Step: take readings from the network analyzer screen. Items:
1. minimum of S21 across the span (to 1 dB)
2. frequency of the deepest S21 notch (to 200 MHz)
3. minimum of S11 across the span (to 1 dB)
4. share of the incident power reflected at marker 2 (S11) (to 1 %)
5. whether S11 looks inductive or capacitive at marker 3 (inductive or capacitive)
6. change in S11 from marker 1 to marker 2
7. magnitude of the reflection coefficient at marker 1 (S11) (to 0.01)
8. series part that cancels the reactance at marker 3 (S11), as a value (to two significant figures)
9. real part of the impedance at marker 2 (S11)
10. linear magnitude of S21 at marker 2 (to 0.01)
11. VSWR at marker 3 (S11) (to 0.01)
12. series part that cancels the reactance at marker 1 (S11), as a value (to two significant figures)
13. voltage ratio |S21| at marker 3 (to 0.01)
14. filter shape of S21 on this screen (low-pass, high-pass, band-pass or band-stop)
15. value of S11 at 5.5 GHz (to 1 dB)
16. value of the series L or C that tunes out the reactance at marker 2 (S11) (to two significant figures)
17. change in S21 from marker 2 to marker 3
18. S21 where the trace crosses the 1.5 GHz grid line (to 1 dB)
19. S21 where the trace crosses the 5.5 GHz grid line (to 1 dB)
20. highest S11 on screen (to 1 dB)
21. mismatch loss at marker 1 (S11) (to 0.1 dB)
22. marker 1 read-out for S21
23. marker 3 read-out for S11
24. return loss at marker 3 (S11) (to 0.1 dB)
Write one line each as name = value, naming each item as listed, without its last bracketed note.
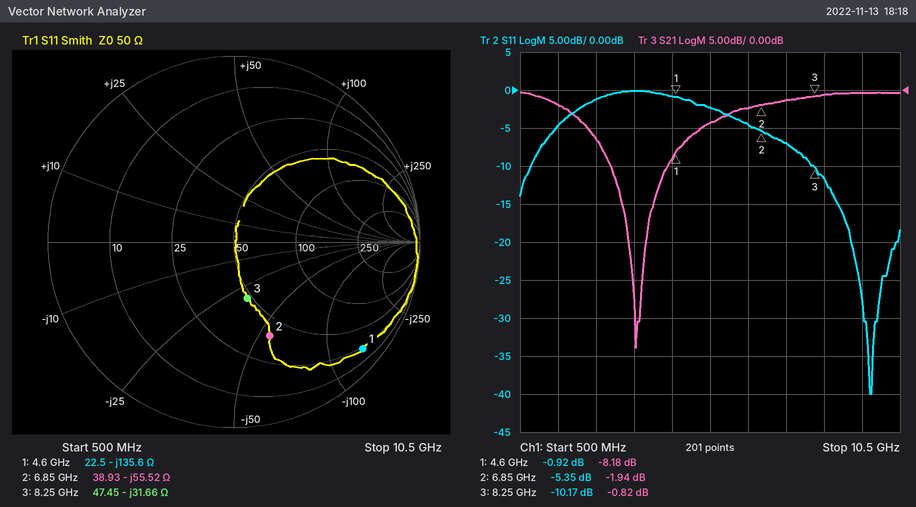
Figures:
minimum of S21 across the span = -34 dB
frequency of the deepest S21 notch = 3.6 GHz
minimum of S11 across the span = -40 dB
share of the incident power reflected at marker 2 (S11) = 29 %
whether S11 looks inductive or capacitive at marker 3 = capacitive
change in S11 from marker 1 to marker 2 = -4.43 dB
magnitude of the reflection coefficient at marker 1 (S11) = 0.90
series part that cancels the reactance at marker 3 (S11), as a value = 610 pH
real part of the impedance at marker 2 = 38.93 Ω
linear magnitude of S21 at marker 2 = 0.80
VSWR at marker 3 (S11) = 1.90
series part that cancels the reactance at marker 1 (S11), as a value = 4.7 nH
voltage ratio |S21| at marker 3 = 0.91
filter shape of S21 on this screen = band-stop
value of S11 at 5.5 GHz = -2 dB
value of the series L or C that tunes out the reactance at marker 2 (S11) = 1.3 nH
change in S21 from marker 2 to marker 3 = 1.12 dB
S21 where the trace crosses the 1.5 GHz grid line = -2 dB
S21 where the trace crosses the 5.5 GHz grid line = -4 dB
highest S11 on screen = 0 dB
mismatch loss at marker 1 (S11) = 7.2 dB
marker 1 read-out for S21 = -8.18 dB
marker 3 read-out for S11 = -10.17 dB
return loss at marker 3 (S11) = 10.2 dB
